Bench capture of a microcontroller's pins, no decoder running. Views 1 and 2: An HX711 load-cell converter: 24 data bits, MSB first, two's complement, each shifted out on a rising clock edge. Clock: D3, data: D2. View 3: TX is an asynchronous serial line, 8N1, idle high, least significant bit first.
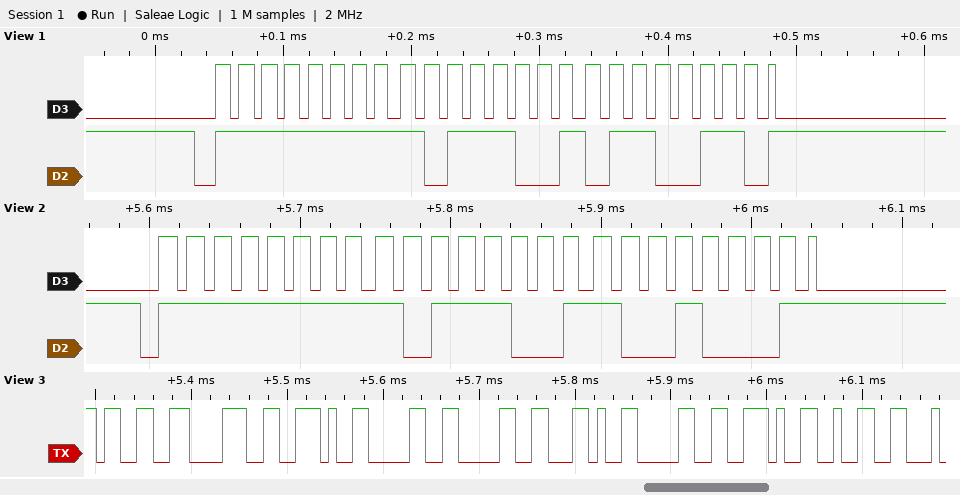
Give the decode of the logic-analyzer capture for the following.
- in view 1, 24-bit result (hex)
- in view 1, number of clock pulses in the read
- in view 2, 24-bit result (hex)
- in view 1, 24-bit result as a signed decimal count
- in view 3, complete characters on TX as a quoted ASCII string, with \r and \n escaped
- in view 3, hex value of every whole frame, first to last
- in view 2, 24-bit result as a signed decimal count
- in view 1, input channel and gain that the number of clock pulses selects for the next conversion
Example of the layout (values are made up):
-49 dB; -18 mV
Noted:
0xFFB966; 25; 0xFFB991; -18074; "38.00,0.2"; 33 38 2E 30 30 2C 30 2E 32; -18031; channel A, gain 128
